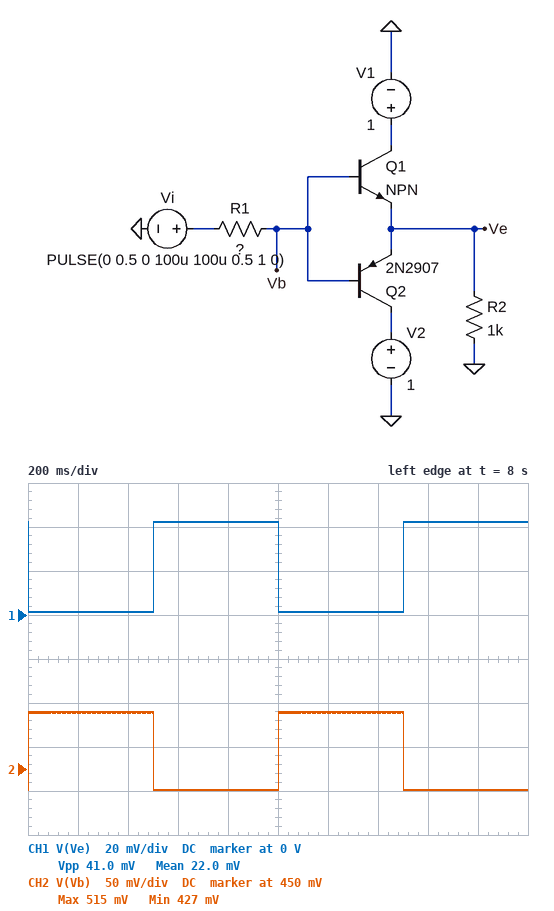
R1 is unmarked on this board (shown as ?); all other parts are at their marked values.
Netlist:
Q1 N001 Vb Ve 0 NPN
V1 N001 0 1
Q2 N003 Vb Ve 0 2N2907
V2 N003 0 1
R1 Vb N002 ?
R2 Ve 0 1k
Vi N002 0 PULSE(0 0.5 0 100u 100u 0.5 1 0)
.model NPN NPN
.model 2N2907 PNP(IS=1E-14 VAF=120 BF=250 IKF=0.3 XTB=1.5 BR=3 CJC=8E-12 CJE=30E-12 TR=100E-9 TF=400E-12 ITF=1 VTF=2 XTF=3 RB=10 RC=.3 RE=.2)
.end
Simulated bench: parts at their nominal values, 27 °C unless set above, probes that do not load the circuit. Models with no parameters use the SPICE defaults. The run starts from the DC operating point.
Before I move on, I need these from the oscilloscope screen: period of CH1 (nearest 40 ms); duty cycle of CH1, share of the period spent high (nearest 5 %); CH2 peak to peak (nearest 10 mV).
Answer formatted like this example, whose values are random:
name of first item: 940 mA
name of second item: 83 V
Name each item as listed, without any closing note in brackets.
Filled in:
period of CH1: 1.00 s
duty cycle of CH1, share of the period spent high: 50 %
CH2 peak to peak: 90 mV
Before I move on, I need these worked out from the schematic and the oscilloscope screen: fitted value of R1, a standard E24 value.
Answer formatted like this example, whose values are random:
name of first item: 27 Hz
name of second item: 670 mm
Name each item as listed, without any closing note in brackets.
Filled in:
fitted value of R1, a standard E24 value: 30 kΩ
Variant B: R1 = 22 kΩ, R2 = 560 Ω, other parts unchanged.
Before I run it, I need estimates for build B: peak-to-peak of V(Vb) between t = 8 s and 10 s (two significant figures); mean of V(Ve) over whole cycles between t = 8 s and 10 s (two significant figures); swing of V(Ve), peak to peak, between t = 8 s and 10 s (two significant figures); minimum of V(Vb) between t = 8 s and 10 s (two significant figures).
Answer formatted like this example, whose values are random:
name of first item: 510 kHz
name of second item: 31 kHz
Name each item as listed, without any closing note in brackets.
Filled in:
peak-to-peak of V(Vb) between t = 8 s and 10 s: 93 mV
mean of V(Ve) over whole cycles between t = 8 s and 10 s: 16 mV
swing of V(Ve), peak to peak, between t = 8 s and 10 s: 31 mV
minimum of V(Vb) between t = 8 s and 10 s: 420 mV
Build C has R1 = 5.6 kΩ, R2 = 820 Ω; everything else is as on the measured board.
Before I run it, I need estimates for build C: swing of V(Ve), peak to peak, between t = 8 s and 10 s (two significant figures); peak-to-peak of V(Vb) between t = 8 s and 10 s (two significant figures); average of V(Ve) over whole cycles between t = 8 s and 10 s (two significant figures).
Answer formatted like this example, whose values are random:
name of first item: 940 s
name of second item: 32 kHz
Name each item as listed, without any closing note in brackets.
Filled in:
swing of V(Ve), peak to peak, between t = 8 s and 10 s: 170 mV
peak-to-peak of V(Vb) between t = 8 s and 10 s: 120 mV
average of V(Ve) over whole cycles between t = 8 s and 10 s: 85 mV
